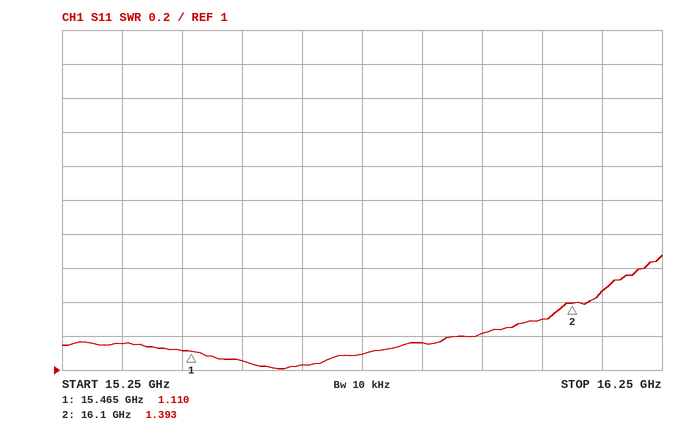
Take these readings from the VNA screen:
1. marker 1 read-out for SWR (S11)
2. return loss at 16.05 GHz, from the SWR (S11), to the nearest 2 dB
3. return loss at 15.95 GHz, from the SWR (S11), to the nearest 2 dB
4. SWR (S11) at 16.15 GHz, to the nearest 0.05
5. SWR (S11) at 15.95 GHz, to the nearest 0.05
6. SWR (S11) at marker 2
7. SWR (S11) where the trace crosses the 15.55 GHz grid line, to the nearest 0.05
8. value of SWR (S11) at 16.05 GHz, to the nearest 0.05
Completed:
1.110
18 dB
20 dB
1.45
1.20
1.393
1.05
1.30
